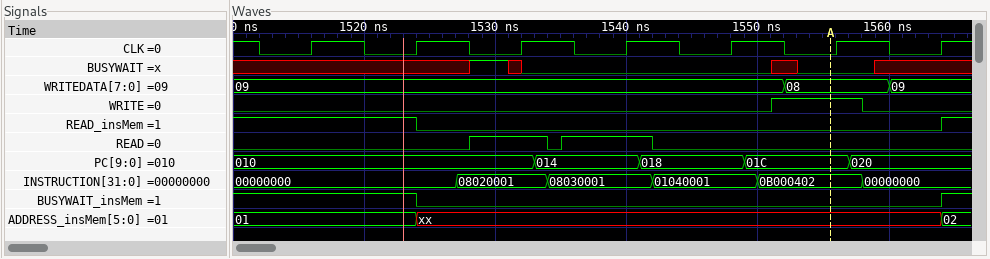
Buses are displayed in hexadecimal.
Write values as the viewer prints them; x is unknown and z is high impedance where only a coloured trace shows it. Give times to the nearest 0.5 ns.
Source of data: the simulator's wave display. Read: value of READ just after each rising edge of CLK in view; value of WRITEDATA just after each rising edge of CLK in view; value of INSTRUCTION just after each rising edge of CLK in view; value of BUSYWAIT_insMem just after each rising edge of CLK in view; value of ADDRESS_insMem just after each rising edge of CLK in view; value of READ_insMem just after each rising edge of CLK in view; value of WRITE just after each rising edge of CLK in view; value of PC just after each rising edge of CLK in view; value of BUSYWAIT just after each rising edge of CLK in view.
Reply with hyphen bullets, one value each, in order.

- 0 0 1 1 0 0 0
- 09, 09, 09, 09, 09, 08, 09
- 00000000, 00000000, 08020001, 08030001, 01040001, 0B000402, 00000000
- 1 0 0 0 0 0 1
- 01, xx, xx, xx, xx, xx, 02
- 1 0 0 0 0 0 1
- 0 0 0 0 0 1 0
- 010, 010, 010, 014, 018, 01C, 020
- x x 0 0 0 0 x
